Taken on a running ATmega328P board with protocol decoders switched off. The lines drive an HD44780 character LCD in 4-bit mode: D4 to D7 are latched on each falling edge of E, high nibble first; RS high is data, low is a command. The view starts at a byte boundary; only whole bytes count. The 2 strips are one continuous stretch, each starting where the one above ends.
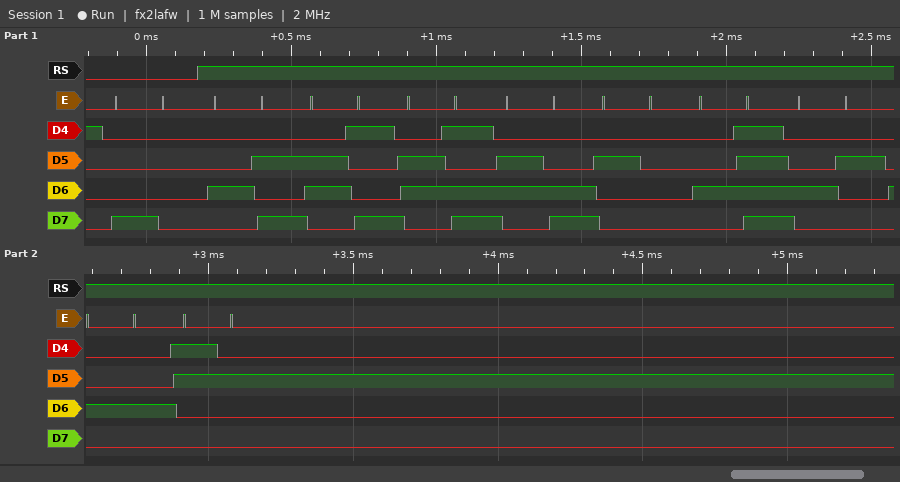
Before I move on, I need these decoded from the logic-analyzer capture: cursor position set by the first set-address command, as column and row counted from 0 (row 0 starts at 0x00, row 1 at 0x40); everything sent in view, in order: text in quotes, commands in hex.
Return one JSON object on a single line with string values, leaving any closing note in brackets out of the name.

{"cursor position set by the first set-address command, as column and row counted from 0": "column 0, row 0", "everything sent in view, in order: text in quotes, commands in hex": "0x80 \"Jiml OBD2\""}
